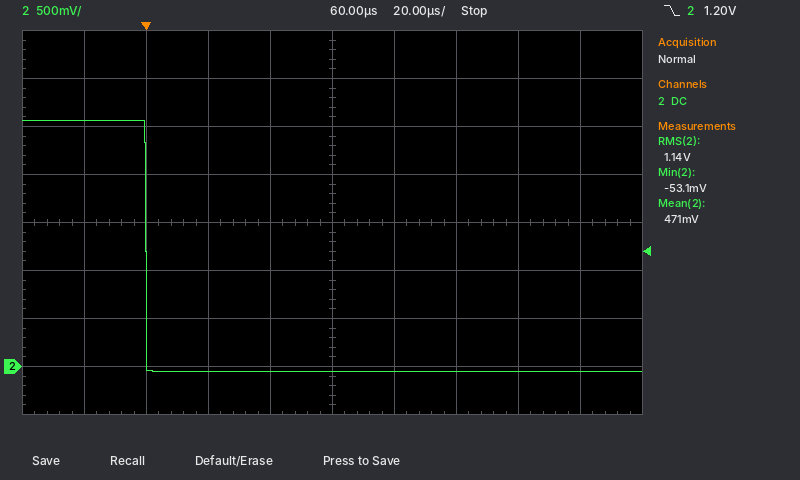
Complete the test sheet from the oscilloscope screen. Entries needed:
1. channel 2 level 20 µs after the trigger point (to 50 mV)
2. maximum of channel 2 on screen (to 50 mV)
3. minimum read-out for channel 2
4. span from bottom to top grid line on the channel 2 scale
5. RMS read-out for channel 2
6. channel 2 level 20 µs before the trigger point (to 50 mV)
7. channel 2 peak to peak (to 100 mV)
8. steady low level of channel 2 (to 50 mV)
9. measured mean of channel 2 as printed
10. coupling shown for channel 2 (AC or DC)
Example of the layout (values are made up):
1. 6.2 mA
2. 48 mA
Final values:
1. -50 mV
2. 2.55 V
3. -53.1 mV
4. 4 V
5. 1.14 V
6. 2.55 V
7. 2.60 V
8. -50 mV
9. 471 mV
10. DC
